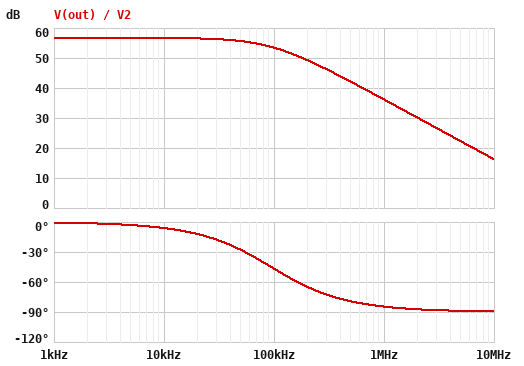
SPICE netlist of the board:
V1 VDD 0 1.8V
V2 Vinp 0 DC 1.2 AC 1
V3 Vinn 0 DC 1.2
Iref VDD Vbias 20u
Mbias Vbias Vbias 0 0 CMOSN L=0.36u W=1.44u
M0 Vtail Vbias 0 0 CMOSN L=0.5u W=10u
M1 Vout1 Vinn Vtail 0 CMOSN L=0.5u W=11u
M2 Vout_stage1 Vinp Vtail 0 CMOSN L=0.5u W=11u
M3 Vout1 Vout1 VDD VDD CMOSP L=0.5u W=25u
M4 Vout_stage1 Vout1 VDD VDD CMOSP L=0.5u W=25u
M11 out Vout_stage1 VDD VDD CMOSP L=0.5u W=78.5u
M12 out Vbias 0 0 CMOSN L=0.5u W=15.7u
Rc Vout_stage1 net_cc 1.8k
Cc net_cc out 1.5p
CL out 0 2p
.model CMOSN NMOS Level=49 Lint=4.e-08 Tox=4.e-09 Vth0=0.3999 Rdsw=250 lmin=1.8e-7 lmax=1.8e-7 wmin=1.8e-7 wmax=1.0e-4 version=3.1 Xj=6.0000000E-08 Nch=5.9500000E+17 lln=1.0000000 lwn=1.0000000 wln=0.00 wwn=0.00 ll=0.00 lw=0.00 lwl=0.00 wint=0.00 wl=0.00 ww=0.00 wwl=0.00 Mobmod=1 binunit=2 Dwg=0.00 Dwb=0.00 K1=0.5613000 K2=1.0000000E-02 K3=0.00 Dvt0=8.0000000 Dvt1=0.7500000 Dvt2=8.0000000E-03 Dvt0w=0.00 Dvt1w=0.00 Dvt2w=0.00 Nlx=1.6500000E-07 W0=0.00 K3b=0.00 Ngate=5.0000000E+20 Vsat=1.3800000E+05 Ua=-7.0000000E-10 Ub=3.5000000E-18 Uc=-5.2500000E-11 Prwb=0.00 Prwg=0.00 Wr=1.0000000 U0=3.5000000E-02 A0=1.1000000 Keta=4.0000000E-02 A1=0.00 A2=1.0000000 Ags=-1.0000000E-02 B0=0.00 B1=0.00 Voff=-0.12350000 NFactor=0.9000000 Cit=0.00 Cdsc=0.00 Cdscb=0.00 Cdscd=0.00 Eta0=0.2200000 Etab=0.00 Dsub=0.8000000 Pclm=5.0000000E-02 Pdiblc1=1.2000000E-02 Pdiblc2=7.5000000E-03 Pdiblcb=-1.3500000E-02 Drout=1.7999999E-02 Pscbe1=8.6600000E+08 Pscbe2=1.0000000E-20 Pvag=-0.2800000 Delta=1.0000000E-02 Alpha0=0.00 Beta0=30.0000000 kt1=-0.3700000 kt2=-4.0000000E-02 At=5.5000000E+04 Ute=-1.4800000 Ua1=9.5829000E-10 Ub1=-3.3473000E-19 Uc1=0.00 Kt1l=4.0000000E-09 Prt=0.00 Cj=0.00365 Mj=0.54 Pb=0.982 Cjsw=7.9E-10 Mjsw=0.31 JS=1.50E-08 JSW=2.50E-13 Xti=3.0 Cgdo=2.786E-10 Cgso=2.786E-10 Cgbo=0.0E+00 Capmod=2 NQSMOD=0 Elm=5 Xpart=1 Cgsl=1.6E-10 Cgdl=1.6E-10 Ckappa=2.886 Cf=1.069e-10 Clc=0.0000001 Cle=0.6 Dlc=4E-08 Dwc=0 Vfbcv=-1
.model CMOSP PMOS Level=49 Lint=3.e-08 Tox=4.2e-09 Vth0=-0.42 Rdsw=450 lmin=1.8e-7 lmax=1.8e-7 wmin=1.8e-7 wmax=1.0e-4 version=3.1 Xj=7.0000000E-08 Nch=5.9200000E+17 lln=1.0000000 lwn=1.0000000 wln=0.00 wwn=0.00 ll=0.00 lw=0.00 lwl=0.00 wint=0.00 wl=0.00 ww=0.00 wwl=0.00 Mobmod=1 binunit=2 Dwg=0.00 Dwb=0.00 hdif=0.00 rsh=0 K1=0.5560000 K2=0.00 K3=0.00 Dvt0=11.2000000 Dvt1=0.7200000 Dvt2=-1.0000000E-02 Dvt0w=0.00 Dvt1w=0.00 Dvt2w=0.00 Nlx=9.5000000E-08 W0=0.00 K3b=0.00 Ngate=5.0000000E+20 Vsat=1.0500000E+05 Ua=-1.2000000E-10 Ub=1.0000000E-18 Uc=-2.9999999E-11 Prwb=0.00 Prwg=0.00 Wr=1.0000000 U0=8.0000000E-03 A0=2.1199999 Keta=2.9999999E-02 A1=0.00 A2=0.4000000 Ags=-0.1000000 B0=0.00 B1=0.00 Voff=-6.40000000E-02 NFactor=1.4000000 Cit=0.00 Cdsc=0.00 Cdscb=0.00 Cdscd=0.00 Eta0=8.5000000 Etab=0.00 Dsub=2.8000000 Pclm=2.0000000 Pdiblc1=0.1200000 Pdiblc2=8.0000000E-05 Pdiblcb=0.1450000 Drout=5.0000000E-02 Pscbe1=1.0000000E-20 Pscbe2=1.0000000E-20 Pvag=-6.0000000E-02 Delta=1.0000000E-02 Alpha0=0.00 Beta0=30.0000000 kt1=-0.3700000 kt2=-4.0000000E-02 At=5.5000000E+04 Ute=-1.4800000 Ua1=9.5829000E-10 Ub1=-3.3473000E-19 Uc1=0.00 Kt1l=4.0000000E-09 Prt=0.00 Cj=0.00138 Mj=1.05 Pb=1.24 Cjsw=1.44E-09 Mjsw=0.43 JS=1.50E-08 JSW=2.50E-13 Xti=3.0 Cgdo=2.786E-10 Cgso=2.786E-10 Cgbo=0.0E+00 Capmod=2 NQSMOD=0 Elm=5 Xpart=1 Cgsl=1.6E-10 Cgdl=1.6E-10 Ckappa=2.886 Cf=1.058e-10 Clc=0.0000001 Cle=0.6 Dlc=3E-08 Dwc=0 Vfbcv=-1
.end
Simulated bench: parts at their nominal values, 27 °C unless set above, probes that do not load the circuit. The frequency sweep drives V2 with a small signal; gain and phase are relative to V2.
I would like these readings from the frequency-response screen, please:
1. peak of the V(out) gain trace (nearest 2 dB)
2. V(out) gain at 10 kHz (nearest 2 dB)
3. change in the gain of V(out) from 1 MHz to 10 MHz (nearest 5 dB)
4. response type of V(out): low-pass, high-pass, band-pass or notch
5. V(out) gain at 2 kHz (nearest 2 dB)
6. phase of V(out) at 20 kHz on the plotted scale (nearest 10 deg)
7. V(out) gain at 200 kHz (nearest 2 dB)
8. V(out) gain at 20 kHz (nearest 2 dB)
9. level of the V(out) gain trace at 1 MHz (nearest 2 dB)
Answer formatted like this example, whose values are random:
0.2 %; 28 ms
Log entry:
56 dB; 56 dB; -20 dB; low-pass; 56 dB; -10 deg; 50 dB; 56 dB; 36 dB
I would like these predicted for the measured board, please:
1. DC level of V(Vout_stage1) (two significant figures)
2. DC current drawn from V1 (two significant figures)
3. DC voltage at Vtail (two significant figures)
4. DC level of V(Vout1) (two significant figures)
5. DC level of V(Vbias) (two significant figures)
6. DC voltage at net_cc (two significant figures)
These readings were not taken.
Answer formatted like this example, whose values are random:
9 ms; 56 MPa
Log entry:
1.1 V; 340 µA; 460 mV; 1.1 V; 690 mV; 1.1 V
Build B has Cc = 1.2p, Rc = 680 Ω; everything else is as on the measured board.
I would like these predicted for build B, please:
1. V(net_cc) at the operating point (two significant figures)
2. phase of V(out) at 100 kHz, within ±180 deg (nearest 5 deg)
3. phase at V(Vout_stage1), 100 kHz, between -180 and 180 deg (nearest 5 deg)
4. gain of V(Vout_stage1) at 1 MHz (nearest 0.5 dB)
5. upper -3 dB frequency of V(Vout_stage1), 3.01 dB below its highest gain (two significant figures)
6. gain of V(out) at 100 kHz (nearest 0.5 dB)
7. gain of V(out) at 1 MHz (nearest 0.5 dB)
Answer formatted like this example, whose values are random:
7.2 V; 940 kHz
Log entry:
1.1 V; -40 deg; 140 deg; 10.0 dB; 120 kHz; 54.5 dB; 38.0 dB
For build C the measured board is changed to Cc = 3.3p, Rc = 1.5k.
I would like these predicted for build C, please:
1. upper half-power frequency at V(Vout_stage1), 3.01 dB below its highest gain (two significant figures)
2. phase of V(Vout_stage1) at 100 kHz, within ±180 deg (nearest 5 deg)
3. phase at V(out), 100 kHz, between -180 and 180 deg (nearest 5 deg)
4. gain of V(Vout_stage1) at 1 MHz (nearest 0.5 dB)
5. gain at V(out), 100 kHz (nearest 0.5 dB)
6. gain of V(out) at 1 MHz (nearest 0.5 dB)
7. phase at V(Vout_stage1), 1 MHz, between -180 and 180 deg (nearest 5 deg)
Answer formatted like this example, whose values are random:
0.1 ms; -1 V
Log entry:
44 kHz; 115 deg; -65 deg; 2.5 dB; 49.0 dB; 29.5 dB; 120 deg
